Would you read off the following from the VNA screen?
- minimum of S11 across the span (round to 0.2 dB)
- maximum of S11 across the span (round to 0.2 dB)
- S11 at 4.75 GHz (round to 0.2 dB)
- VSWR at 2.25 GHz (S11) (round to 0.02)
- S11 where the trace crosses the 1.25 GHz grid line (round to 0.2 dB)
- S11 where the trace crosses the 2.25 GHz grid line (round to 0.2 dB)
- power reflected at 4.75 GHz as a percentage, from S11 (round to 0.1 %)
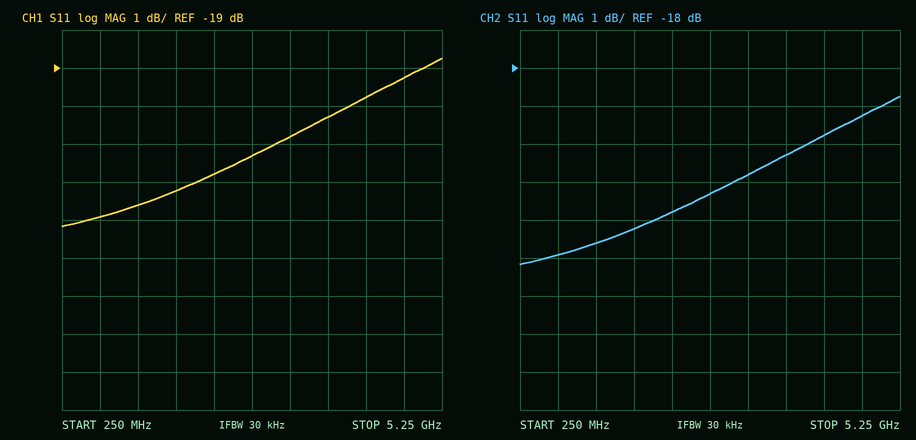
-23.2 dB
-18.8 dB
-19.2 dB
1.18
-22.6 dB
-21.8 dB
1.2 %
